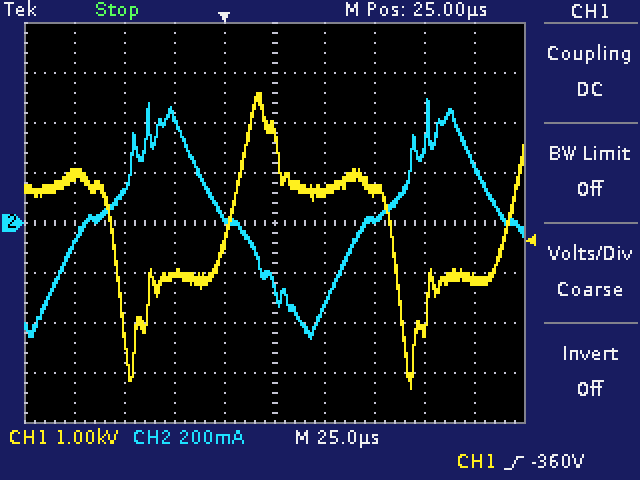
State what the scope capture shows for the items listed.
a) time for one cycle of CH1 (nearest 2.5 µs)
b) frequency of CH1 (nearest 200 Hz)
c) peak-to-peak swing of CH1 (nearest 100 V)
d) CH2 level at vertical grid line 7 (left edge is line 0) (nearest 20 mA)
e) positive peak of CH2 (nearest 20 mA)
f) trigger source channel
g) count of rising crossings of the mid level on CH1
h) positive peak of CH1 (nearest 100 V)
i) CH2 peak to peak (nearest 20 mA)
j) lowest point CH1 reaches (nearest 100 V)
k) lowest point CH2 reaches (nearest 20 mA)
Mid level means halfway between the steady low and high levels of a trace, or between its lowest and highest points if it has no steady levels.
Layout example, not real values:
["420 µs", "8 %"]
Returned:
["140.0 µs", "7.2 kHz", "5.9 kV", "20 mA", "500 mA", "CH1", "2", "2.6 kV", "960 mA", "-3.3 kV", "-460 mA"]
